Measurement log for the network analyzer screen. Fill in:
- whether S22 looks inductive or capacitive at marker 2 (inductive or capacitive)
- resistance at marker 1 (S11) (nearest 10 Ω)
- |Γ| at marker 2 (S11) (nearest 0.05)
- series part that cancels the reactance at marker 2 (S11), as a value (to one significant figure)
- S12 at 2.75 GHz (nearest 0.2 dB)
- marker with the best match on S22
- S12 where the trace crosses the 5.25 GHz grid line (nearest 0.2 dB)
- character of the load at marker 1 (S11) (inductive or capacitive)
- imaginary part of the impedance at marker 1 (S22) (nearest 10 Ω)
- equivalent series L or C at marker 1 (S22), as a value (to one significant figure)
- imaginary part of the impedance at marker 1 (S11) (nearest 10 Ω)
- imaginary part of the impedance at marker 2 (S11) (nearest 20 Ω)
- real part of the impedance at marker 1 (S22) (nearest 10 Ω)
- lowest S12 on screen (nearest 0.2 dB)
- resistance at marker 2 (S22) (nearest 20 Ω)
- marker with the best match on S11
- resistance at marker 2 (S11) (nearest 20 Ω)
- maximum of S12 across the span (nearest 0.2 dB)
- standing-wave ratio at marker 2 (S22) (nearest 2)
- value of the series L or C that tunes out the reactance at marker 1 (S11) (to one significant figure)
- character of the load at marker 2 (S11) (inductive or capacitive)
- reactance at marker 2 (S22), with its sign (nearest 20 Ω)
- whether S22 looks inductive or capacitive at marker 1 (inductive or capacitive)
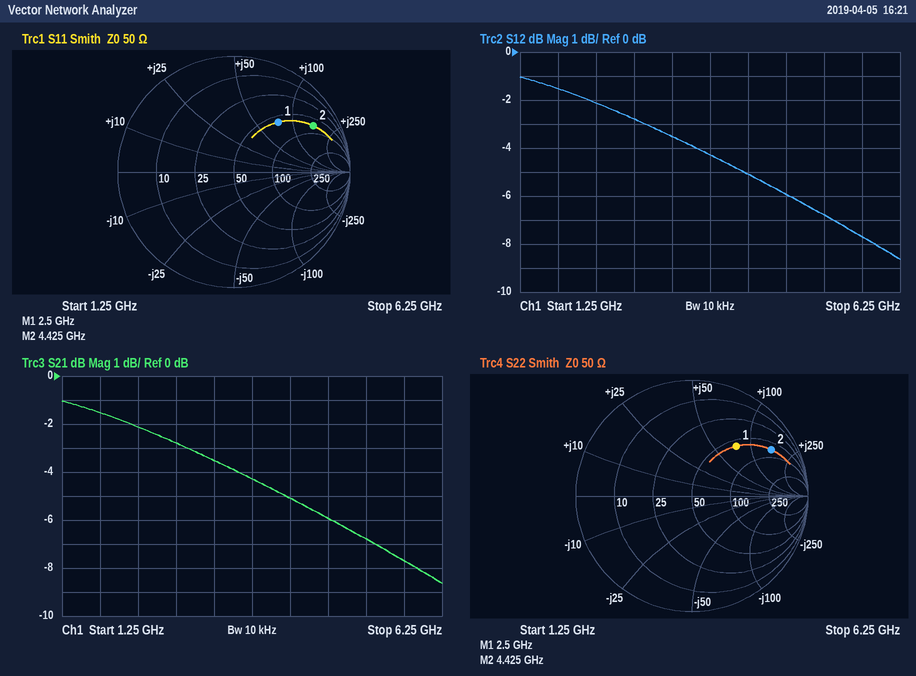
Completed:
inductive
60 Ω
0.80
200 fF
-2.8 dB
marker 1
-6.8 dB
inductive
+80 Ω
5 nH
+80 Ω
+160 Ω
60 Ω
-8.6 dB
80 Ω
marker 1
80 Ω
-1.0 dB
8
800 fF
inductive
+160 Ω
inductive
